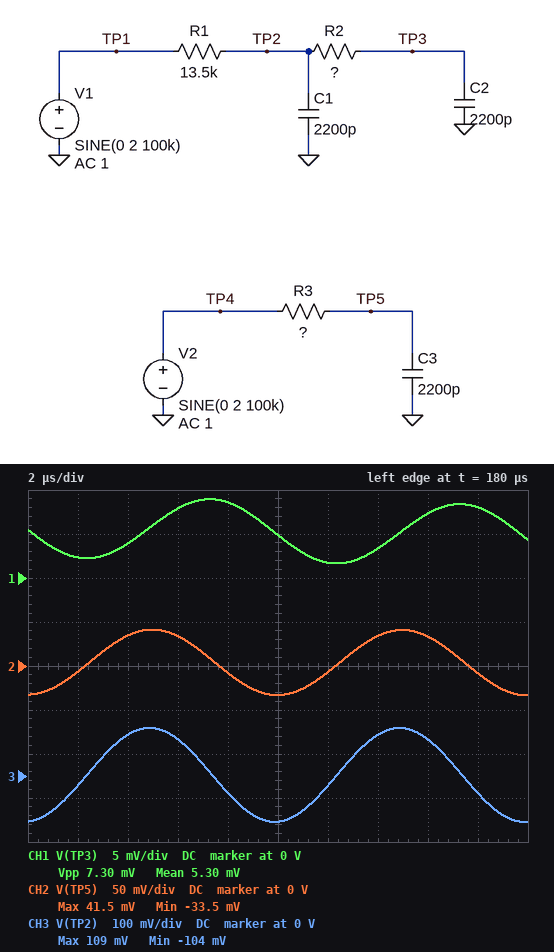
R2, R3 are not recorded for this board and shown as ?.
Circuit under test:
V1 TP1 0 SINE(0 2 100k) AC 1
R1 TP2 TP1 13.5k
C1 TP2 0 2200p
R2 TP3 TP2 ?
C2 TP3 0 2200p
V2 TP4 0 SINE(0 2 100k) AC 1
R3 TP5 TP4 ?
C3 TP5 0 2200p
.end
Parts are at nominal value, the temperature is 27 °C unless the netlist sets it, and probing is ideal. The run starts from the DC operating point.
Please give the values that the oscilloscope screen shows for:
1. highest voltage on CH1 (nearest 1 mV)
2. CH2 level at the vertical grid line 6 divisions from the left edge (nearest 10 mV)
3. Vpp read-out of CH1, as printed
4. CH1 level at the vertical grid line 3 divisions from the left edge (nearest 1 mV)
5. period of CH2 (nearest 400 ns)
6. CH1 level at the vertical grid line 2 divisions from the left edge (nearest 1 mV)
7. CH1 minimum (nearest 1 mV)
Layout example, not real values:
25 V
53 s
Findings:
9 mV
-10 mV
7.30 mV
8 mV
10.0 µs
4 mV
2 mV
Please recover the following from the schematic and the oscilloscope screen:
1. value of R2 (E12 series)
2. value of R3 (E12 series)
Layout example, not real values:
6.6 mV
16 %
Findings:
22 kΩ
39 kΩ
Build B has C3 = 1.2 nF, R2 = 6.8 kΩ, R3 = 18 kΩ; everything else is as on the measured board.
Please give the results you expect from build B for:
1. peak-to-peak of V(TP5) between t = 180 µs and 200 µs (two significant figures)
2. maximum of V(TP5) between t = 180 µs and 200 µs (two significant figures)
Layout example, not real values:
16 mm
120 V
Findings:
290 mV
150 mV
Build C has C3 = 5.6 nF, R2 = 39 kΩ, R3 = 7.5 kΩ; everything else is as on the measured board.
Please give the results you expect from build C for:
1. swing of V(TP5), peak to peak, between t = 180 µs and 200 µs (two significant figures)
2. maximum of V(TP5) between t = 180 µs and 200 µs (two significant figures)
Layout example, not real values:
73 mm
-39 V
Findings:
150 mV
77 mV
